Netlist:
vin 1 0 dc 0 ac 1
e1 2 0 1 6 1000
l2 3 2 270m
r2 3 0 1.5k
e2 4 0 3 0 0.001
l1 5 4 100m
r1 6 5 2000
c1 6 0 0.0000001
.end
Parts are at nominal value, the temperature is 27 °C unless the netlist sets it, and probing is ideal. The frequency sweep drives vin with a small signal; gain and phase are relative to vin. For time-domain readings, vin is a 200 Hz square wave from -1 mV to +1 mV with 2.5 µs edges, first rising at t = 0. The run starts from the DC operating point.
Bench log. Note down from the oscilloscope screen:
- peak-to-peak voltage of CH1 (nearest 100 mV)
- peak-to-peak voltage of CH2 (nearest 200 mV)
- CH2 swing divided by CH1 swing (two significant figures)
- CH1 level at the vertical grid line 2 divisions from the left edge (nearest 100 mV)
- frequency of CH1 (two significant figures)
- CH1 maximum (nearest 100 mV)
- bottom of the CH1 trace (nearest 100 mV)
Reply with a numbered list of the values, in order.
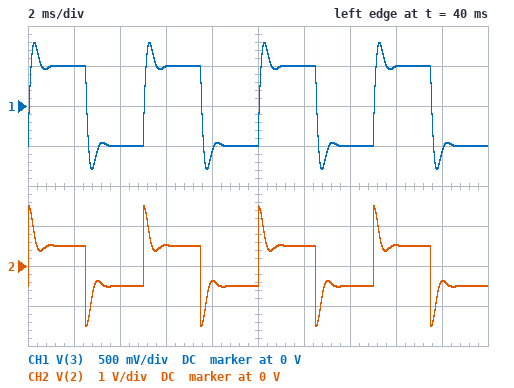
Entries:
1. 1.6 V
2. 3.0 V
3. 1.9
4. -500 mV
5. 200 Hz
6. 800 mV
7. -800 mV
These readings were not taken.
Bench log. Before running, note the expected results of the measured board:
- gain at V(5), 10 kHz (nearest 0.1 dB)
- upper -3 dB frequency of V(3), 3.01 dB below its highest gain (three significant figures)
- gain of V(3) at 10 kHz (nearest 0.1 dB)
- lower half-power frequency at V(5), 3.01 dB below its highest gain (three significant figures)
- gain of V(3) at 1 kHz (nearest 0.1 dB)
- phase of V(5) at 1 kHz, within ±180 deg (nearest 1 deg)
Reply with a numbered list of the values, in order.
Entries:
1. -31.2 dB
2. 1.88 kHz
3. 38.9 dB
4. 441 Hz
5. 57.1 dB
6. -33 deg
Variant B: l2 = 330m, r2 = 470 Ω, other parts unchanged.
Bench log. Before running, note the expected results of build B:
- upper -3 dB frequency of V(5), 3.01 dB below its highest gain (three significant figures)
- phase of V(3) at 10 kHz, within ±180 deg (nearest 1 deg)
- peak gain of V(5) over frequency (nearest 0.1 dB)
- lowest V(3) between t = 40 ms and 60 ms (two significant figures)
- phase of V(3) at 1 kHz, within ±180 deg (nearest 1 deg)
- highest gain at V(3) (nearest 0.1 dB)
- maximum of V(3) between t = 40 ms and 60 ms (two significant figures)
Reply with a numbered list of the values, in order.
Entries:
1. 786 Hz
2. -89 deg
3. -6.0 dB
4. -510 mV
5. -71 deg
6. 54.0 dB
7. 510 mV
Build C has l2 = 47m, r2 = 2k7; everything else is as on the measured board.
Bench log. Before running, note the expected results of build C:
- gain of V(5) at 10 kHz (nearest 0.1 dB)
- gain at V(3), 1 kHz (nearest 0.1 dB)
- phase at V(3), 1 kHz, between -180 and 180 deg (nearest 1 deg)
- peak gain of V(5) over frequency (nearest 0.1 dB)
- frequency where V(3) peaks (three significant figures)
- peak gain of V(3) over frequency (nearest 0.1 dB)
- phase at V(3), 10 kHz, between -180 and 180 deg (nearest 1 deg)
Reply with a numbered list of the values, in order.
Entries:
1. -13.4 dB
2. 57.0 dB
3. 22 deg
4. 1.1 dB
5. 2.60 kHz
6. 61.1 dB
7. -48 deg
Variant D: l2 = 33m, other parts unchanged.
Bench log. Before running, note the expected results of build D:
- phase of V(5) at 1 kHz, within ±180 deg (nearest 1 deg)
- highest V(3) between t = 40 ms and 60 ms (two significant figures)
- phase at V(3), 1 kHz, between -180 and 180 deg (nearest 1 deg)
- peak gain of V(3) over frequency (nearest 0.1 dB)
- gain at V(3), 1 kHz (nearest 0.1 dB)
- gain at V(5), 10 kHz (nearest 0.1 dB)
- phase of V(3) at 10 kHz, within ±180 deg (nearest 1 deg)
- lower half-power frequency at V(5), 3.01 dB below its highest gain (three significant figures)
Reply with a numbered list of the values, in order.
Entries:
1. 8 deg
2. 1.3 V
3. 21 deg
4. 61.1 dB
5. 57.0 dB
6. -14.7 dB
7. -55 deg
8. 977 Hz
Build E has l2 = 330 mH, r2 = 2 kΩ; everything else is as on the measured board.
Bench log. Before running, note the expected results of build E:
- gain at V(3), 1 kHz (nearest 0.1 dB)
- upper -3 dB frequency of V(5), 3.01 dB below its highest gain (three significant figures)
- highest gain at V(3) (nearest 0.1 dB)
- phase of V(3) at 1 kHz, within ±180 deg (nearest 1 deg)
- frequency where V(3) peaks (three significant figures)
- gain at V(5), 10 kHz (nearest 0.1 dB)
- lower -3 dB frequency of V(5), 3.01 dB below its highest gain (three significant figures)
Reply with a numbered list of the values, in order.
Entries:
1. 57.3 dB
2. 1.84 kHz
3. 57.5 dB
4. -17 deg
5. 1.17 kHz
6. -30.5 dB
7. 493 Hz
